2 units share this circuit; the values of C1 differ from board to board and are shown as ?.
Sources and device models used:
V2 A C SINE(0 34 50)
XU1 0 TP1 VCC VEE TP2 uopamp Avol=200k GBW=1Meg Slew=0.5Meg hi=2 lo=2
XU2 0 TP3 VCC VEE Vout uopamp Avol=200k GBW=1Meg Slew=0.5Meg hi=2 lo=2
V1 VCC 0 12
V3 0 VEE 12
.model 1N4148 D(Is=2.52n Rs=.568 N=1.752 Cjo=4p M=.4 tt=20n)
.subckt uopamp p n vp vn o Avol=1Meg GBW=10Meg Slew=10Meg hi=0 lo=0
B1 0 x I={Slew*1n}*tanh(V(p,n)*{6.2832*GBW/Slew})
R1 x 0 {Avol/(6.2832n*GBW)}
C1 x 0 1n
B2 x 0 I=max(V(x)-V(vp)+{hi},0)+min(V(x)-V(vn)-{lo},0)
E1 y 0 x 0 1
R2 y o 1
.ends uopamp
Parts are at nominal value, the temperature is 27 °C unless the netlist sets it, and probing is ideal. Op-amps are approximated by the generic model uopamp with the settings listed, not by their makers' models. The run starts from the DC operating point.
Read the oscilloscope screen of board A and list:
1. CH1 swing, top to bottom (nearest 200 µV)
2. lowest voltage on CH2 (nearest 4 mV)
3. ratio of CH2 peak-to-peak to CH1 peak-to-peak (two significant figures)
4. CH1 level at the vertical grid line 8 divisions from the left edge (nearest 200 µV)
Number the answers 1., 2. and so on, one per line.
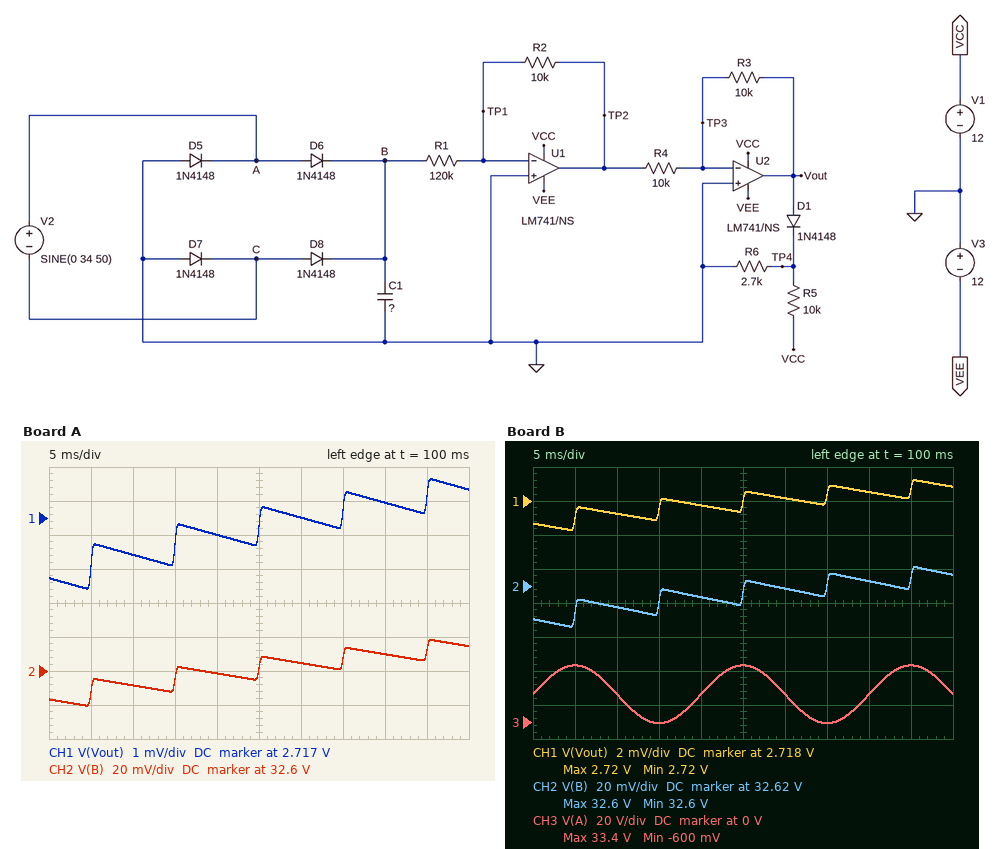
1. 3.2 mV
2. 32.580 V
3. 12
4. 2.7174 V
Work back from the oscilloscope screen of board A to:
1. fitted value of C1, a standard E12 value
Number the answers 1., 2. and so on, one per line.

1. 330 µF
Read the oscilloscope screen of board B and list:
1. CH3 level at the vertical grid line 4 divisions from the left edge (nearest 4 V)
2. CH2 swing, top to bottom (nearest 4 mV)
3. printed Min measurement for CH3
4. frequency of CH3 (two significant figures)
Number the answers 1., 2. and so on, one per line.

1. 16 V
2. 36 mV
3. -600 mV
4. 50 Hz
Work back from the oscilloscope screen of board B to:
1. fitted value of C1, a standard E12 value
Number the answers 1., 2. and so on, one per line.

1. 270 µF
